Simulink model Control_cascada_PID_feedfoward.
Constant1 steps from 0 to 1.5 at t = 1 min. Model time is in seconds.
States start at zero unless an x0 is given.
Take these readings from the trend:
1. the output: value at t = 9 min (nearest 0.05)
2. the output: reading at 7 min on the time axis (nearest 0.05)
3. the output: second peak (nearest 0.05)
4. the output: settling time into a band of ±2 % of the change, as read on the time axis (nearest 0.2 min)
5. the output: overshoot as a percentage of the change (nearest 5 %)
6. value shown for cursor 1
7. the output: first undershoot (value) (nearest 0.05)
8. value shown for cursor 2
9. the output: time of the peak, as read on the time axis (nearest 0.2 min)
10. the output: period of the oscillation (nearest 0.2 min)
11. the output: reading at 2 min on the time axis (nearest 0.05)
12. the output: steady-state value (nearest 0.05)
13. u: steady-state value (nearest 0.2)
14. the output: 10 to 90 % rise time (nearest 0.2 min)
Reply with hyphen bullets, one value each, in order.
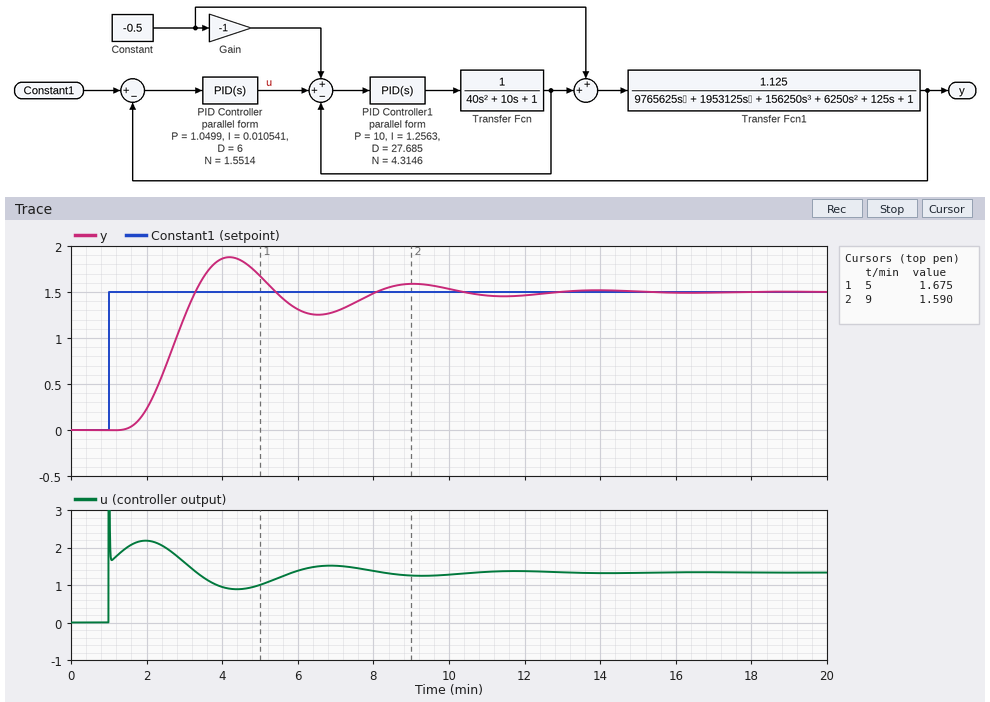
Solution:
- 1.60
- 1.30
- 1.60
- 12.2 min
- 25 %
- 1.675
- 1.25
- 1.590
- 4.2 min
- 4.8 min
- 0.25
- 1.50
- 1.4
- 1.2 min
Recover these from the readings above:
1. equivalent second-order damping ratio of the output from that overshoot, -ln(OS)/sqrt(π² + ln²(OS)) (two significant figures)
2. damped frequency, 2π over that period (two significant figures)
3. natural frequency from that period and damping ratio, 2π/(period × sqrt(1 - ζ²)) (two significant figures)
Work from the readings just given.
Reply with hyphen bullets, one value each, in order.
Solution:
- 0.40
- 1.3 rad/min
- 1.4 rad/min
